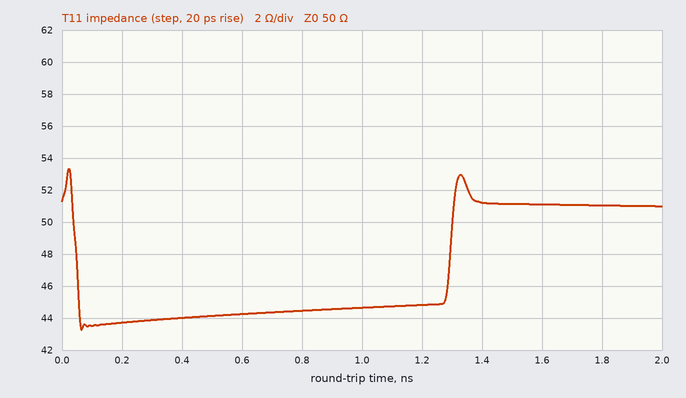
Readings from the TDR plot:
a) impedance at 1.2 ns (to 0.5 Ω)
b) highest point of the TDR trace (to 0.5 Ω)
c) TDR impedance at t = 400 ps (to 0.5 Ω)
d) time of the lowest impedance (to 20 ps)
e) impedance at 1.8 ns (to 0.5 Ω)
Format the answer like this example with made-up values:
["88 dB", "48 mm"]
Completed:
["45.0 Ω", "53.5 Ω", "44.0 Ω", "60 ps", "51.0 Ω"]
